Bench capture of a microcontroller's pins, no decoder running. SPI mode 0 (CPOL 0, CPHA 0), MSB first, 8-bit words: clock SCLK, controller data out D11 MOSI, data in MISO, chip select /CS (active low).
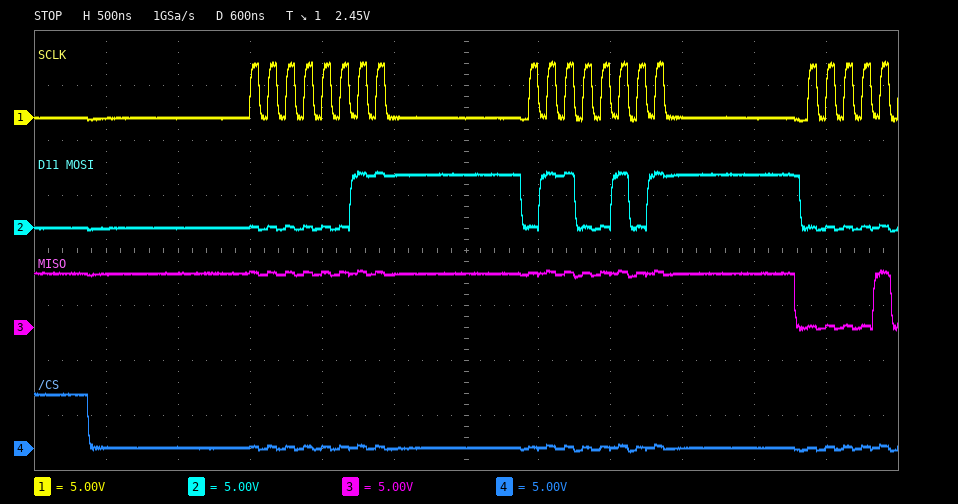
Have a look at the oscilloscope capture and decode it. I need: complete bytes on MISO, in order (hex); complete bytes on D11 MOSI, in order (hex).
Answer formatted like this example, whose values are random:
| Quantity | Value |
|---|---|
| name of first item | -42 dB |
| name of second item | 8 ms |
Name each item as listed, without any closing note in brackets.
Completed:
| Quantity | Value |
|---|---|
| complete bytes on MISO, in order | 0xFF 0xFF |
| complete bytes on D11 MOSI, in order | 0x03 0x65 |
